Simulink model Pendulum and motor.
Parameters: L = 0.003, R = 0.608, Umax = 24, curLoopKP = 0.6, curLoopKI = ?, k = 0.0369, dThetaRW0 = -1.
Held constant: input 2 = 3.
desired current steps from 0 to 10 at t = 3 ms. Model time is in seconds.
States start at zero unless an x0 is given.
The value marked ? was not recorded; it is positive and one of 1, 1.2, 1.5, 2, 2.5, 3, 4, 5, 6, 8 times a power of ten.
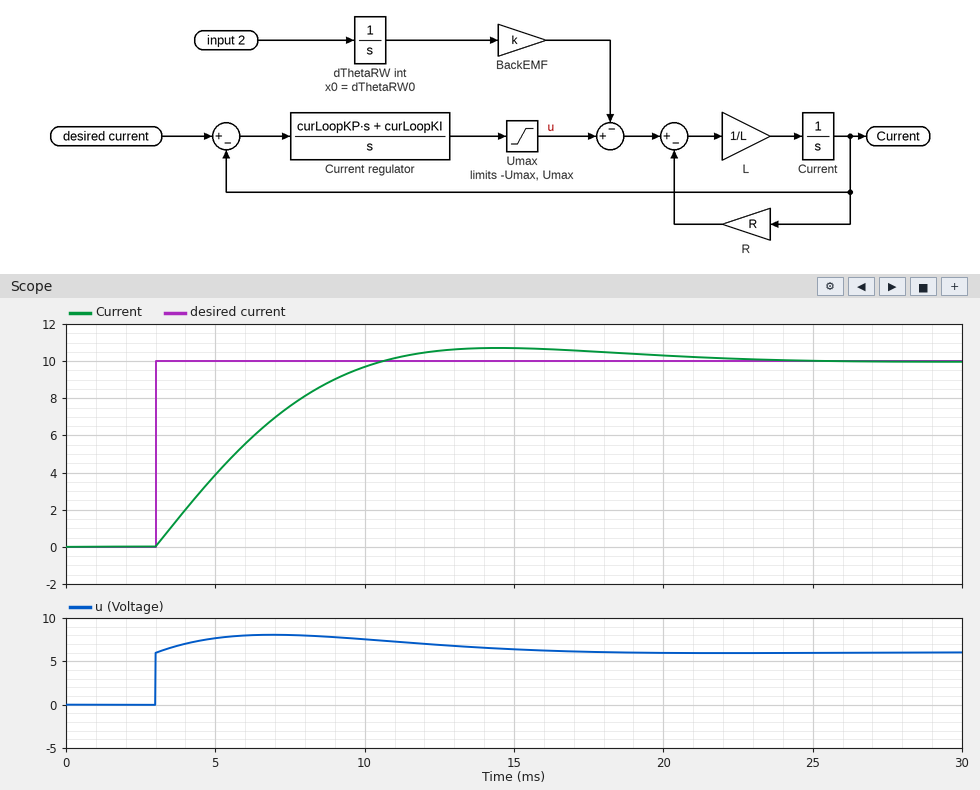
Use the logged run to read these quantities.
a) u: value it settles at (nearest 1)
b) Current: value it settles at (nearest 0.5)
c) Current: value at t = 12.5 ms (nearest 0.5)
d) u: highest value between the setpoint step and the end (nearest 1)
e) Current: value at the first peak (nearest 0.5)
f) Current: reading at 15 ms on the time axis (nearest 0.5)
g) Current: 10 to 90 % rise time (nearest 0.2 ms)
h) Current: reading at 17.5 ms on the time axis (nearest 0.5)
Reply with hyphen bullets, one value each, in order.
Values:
- 6
- 10.0
- 10.5
- 8
- 10.5
- 10.5
- 5.4 ms
- 10.5
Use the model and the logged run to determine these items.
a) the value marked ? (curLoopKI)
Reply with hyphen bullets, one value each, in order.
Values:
- 250
